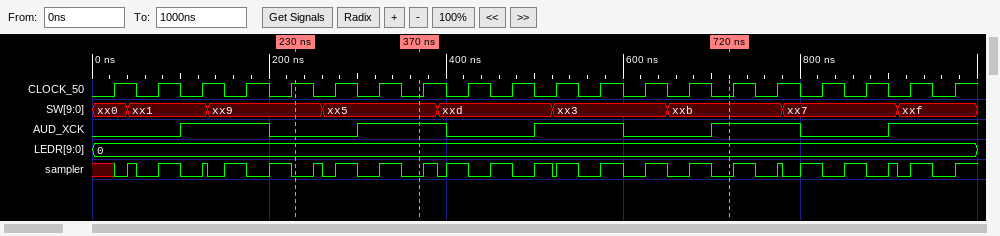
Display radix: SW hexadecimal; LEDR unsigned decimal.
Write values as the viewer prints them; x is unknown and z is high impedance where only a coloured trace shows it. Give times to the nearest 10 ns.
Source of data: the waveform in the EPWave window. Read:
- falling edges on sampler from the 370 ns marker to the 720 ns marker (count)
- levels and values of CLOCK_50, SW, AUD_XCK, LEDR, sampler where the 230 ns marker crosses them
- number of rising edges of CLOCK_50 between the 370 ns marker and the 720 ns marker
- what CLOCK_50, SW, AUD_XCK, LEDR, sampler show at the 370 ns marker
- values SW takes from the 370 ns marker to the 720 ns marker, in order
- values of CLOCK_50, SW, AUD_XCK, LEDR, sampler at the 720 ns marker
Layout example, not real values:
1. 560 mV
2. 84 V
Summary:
1. 8
2. CLOCK_50=1, SW=xx9, AUD_XCK=0, LEDR=0, sampler=0
3. 7
4. CLOCK_50=0, SW=xx5, AUD_XCK=1, LEDR=0, sampler=0
5. xx5, xxd, xx3, xxb
6. CLOCK_50=0, SW=xxb, AUD_XCK=1, LEDR=0, sampler=0
